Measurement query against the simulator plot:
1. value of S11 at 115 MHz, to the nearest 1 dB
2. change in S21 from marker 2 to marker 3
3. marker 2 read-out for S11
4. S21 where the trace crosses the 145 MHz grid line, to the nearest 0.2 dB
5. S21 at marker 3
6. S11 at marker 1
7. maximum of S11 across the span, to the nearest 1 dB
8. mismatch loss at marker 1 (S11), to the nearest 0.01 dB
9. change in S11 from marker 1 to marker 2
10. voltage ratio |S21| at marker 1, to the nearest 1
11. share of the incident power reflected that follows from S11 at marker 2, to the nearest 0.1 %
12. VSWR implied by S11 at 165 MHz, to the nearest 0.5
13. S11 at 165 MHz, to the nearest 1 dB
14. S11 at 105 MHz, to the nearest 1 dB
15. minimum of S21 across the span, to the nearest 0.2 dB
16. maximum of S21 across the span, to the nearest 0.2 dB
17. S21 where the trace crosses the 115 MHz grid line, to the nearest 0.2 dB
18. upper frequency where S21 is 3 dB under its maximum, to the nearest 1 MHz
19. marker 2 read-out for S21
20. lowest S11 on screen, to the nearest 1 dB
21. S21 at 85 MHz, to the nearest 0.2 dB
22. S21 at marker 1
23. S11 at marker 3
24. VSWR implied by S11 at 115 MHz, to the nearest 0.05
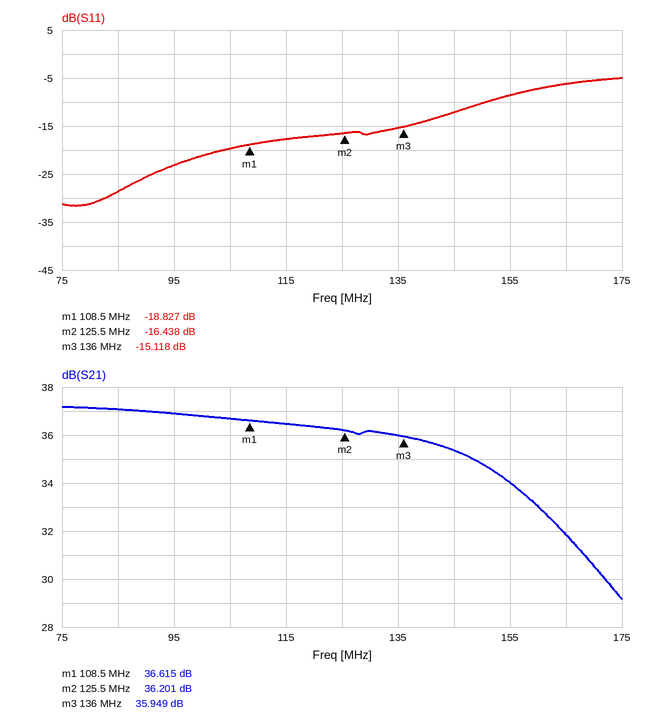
-18 dB
-0.252 dB
-16.438 dB
35.4 dB
35.949 dB
-18.827 dB
-5 dB
0.06 dB
2.389 dB
68
2.3 %
3.0
-6 dB
-20 dB
29.2 dB
37.2 dB
36.4 dB
154 MHz
36.201 dB
-32 dB
37.0 dB
36.615 dB
-15.118 dB
1.30
